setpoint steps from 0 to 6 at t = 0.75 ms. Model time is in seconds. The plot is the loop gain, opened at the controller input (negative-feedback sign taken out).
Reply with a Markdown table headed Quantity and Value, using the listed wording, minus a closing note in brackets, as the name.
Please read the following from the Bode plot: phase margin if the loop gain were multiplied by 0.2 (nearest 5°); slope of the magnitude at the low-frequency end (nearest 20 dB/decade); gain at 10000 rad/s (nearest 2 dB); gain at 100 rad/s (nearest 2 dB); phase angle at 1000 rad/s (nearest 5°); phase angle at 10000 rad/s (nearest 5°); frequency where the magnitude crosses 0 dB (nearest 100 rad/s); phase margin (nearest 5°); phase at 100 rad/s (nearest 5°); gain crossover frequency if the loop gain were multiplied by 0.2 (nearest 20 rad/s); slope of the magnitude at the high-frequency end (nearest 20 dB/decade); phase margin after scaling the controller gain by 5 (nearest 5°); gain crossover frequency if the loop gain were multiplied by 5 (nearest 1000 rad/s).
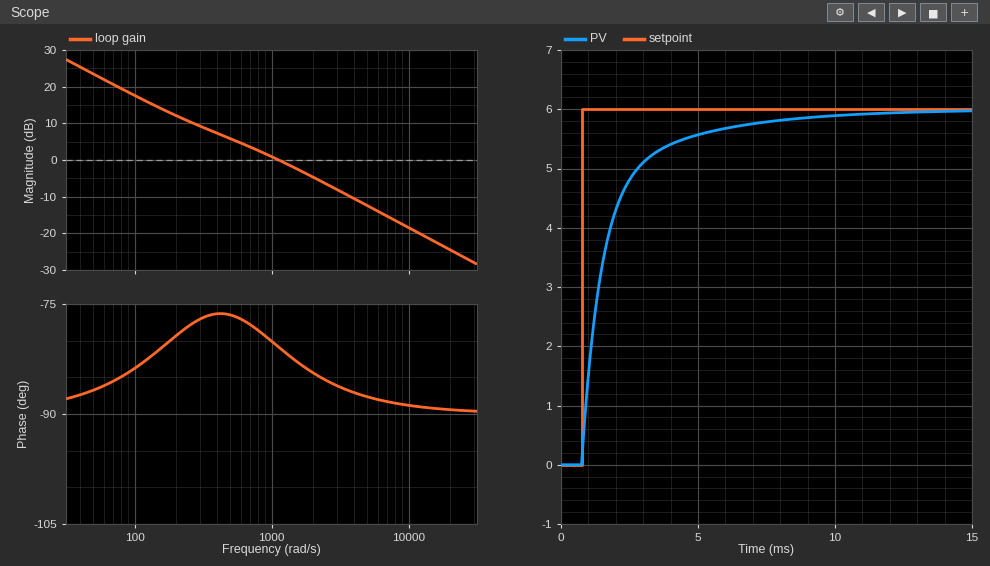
| Quantity | Value |
|---|---|
| phase margin if the loop gain were multiplied by 0.2 | 100° |
| slope of the magnitude at the low-frequency end | -20 dB/decade |
| gain at 10000 rad/s | -18 dB |
| gain at 100 rad/s | 18 dB |
| phase angle at 1000 rad/s | -80° |
| phase angle at 10000 rad/s | -90° |
| frequency where the magnitude crosses 0 dB | 1100 rad/s |
| phase margin | 100° |
| phase at 100 rad/s | -85° |
| gain crossover frequency if the loop gain were multiplied by 0.2 | 160 rad/s |
| slope of the magnitude at the high-frequency end | -20 dB/decade |
| phase margin after scaling the controller gain by 5 | 90° |
| gain crossover frequency if the loop gain were multiplied by 5 | 6000 rad/s |
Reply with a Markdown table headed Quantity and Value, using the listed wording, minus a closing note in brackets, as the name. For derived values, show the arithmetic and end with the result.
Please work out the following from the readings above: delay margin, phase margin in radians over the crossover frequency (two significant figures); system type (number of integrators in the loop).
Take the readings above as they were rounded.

| Quantity | Value |
|---|---|
| delay margin, phase margin in radians over the crossover frequency | 100 × π / 180 / 1100 = 0.0016 s |
| system type | 1 |
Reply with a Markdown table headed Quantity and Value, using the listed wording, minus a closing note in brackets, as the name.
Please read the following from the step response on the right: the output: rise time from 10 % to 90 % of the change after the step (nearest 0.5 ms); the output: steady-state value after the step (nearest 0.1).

| Quantity | Value |
|---|---|
| the output: rise time from 10 % to 90 % of the change after the step | 3.0 ms |
| the output: steady-state value after the step | 6.0 |
